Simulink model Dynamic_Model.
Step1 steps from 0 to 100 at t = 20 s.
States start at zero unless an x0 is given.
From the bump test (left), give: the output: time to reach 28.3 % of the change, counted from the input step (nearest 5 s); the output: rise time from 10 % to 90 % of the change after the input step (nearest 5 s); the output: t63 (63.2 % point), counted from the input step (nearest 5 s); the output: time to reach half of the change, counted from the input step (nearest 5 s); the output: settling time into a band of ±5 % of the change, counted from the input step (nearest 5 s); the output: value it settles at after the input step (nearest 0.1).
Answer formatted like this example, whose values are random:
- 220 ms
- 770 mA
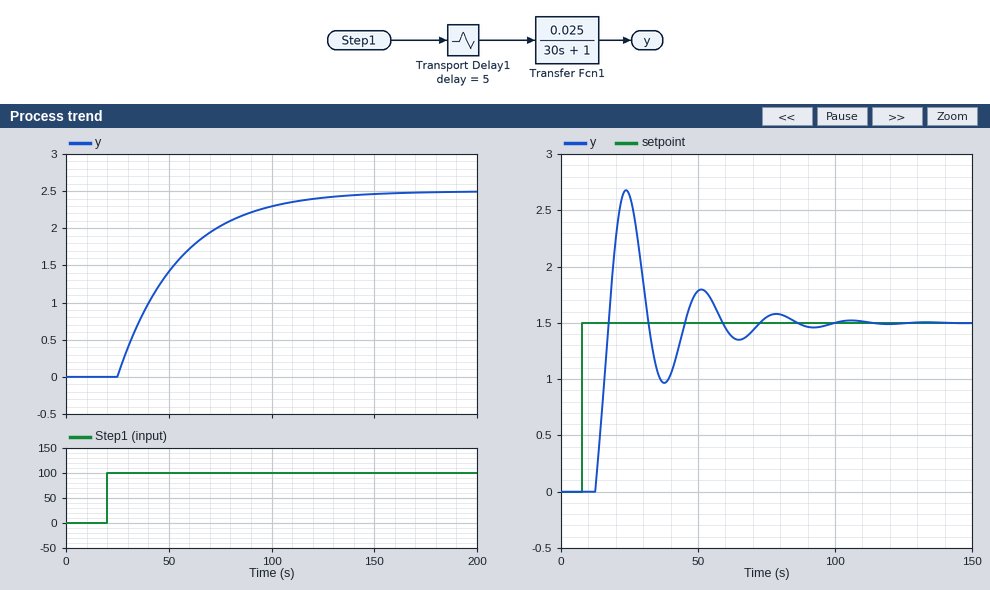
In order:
- 15 s
- 65 s
- 35 s
- 25 s
- 95 s
- 2.5
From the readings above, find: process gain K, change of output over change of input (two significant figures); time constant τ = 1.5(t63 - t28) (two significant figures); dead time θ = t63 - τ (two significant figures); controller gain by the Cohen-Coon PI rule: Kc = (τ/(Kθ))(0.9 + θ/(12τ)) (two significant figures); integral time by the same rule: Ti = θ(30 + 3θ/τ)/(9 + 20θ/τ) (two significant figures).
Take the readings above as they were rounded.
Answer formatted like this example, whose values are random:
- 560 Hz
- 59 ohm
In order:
- 0.025
- 30 s
- 5.0 s
- 220
- 12 s
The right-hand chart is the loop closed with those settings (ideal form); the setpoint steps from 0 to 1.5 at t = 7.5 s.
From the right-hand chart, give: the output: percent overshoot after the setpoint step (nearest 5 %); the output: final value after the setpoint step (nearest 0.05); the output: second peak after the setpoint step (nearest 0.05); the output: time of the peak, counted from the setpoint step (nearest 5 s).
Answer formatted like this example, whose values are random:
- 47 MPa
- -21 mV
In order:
- 80 %
- 1.50
- 1.80
- 15 s
